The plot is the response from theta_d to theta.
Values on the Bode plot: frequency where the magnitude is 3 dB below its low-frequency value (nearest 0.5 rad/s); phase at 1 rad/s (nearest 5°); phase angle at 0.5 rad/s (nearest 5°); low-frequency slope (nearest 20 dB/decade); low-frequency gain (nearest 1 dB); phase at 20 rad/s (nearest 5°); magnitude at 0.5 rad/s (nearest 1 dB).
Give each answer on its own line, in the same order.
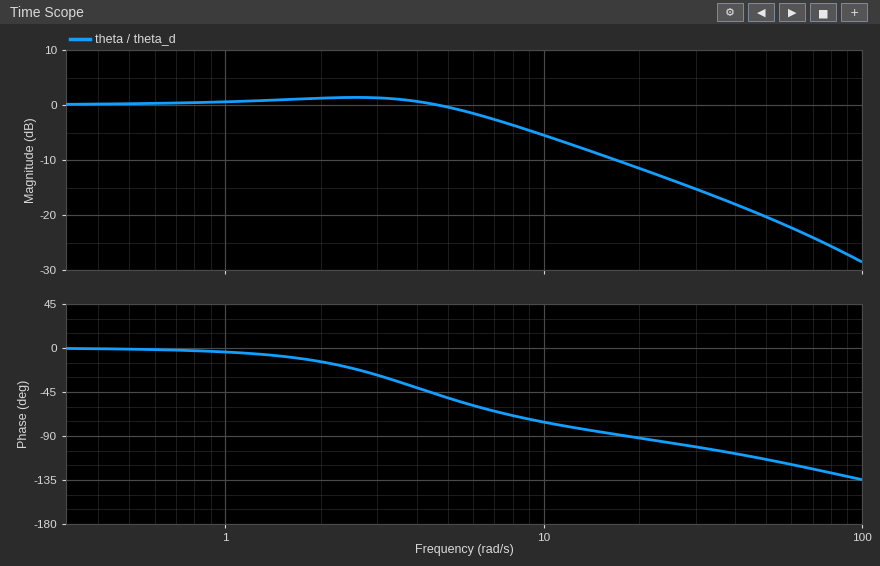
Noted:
7.0 rad/s
-5°
0°
0 dB/decade
0 dB
-90°
0 dB
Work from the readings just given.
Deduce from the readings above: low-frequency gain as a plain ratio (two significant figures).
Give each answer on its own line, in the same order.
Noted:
1.0
